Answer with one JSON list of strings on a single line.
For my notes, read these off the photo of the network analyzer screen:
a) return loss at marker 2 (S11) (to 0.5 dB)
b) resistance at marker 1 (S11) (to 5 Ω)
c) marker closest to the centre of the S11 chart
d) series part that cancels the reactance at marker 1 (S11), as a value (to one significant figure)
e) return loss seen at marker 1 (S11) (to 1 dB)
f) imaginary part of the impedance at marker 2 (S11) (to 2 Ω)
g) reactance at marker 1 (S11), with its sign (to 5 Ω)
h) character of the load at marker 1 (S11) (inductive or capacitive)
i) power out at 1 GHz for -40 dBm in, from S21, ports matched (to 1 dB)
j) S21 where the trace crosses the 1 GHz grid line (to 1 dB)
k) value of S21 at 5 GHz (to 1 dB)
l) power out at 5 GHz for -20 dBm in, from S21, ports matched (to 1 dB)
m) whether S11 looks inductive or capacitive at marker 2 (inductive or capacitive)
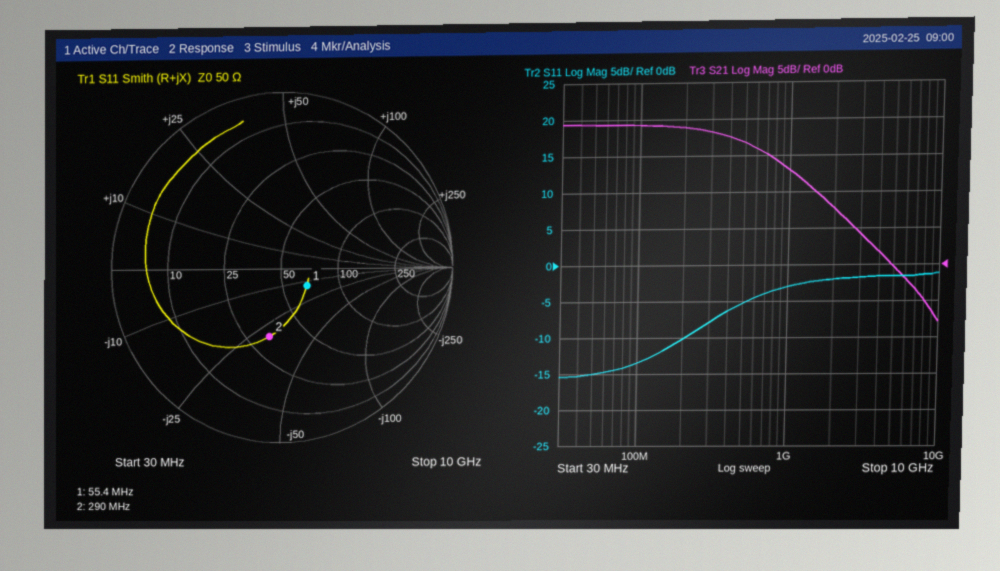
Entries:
["8.0 dB", "65 Ω", "marker 1", "40 nH", "15 dB", "-30 Ω", "-15 Ω", "capacitive", "-27 dBm", "13 dB", "0 dB", "-20 dBm", "capacitive"]
